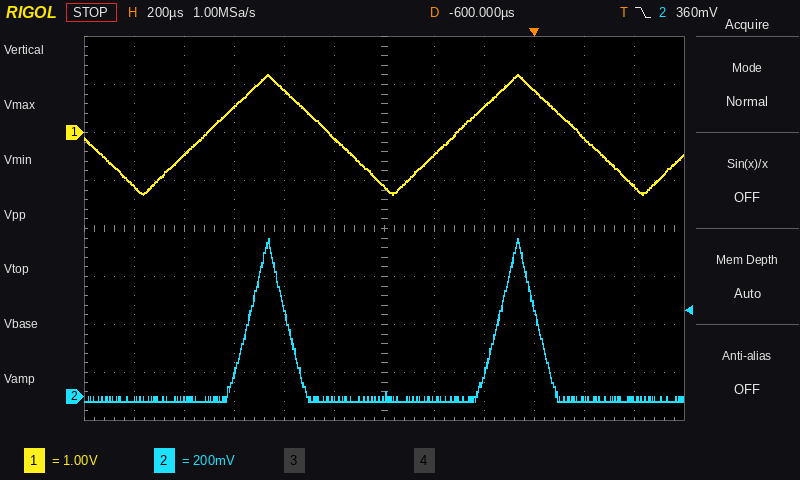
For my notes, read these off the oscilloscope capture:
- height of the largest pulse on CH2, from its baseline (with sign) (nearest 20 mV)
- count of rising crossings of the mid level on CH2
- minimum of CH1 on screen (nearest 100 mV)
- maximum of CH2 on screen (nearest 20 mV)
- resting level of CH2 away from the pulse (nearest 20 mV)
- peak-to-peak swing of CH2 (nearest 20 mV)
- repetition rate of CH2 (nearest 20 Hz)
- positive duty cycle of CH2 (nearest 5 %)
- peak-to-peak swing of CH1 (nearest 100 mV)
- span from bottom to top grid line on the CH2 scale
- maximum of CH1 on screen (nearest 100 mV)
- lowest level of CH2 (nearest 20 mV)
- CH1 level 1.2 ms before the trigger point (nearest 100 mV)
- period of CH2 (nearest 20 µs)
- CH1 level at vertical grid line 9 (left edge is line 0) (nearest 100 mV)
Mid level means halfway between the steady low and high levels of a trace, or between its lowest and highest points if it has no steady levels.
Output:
+680 mV
2
-1.3 V
660 mV
-20 mV
680 mV
1.00 kHz
15 %
2.5 V
1.6 V
1.2 V
-20 mV
500 mV
1.00 ms
900 mV
